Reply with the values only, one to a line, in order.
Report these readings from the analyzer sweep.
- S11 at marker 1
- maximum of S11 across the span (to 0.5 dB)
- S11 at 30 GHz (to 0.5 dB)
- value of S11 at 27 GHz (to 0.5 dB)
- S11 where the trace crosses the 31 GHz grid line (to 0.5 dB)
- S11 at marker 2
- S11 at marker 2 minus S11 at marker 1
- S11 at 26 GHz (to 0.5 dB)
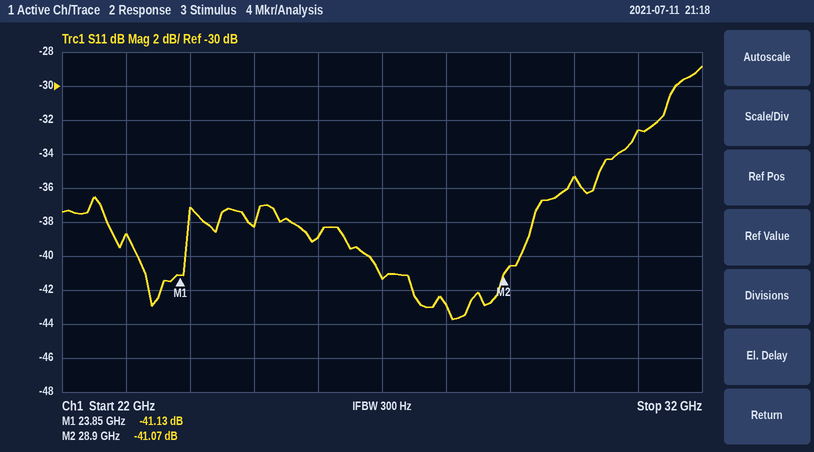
-41.13 dB
-29.0 dB
-35.5 dB
-41.5 dB
-32.5 dB
-41.07 dB
0.06 dB
-39.0 dB
